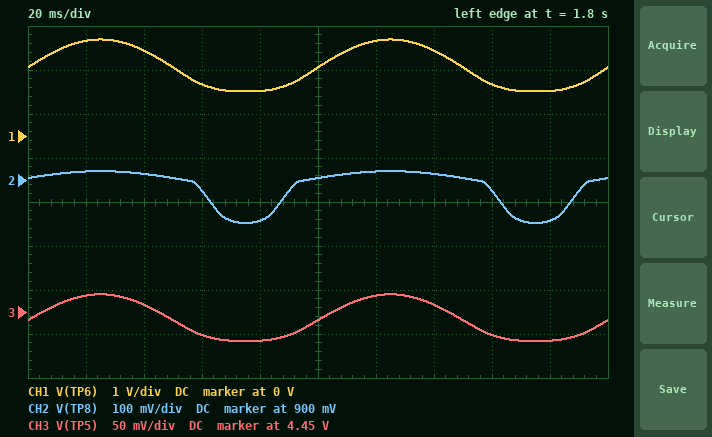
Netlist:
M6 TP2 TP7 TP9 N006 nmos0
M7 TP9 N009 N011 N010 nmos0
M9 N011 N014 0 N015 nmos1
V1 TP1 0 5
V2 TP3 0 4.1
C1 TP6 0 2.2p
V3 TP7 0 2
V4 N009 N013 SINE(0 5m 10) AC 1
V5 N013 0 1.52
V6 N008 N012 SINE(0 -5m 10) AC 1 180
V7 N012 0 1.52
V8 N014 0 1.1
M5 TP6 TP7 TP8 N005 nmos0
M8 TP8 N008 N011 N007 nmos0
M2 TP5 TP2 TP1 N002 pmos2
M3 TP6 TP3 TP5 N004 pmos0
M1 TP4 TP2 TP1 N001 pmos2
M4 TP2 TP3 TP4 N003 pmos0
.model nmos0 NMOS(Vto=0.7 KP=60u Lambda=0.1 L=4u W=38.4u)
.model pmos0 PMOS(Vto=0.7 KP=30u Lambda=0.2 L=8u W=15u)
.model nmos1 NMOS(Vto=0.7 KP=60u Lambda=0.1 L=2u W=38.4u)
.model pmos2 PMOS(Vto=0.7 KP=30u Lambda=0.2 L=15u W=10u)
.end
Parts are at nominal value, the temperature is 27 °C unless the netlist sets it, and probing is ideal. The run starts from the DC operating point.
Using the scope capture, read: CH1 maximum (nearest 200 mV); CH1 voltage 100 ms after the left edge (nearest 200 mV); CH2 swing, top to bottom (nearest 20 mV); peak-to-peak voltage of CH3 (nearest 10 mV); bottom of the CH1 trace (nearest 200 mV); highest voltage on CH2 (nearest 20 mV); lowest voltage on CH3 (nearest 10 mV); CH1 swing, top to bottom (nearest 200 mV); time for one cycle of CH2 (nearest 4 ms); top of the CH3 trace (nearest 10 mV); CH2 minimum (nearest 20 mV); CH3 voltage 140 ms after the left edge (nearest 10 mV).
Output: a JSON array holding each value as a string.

["2.2 V", "1.6 V", "120 mV", "50 mV", "1.0 V", "920 mV", "4.42 V", "1.2 V", "100 ms", "4.47 V", "800 mV", "4.46 V"]
